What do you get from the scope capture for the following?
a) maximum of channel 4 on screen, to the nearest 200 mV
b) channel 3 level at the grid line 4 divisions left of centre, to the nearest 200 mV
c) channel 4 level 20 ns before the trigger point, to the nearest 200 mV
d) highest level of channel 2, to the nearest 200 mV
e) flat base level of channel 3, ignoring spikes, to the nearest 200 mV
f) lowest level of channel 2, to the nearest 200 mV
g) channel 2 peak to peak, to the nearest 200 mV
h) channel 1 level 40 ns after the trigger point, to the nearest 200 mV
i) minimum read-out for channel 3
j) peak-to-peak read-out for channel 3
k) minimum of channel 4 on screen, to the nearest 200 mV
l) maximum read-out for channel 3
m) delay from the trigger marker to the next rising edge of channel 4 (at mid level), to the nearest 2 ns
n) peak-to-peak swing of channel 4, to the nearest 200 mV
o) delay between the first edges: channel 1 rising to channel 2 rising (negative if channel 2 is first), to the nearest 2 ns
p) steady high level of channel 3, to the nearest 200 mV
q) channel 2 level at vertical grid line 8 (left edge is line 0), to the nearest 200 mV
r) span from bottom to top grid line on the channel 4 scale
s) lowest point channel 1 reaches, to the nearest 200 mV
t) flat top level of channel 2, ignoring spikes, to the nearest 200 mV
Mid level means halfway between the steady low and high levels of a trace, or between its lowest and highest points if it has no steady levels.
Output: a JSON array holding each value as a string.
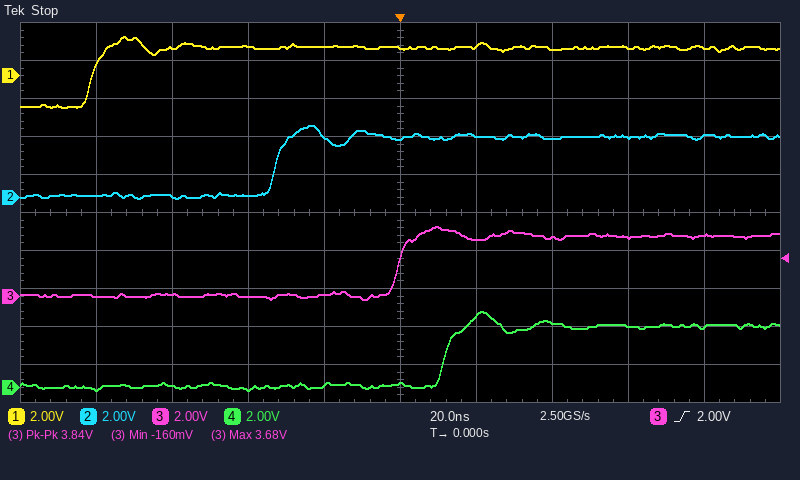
["4.0 V", "0.0 V", "200 mV", "3.8 V", "0.0 V", "0.0 V", "3.8 V", "1.4 V", "-160 mV", "3.84 V", "-200 mV", "3.68 V", "12 ns", "4.2 V", "+48 ns", "3.2 V", "3.2 V", "20 V", "-1.6 V", "3.2 V"]
